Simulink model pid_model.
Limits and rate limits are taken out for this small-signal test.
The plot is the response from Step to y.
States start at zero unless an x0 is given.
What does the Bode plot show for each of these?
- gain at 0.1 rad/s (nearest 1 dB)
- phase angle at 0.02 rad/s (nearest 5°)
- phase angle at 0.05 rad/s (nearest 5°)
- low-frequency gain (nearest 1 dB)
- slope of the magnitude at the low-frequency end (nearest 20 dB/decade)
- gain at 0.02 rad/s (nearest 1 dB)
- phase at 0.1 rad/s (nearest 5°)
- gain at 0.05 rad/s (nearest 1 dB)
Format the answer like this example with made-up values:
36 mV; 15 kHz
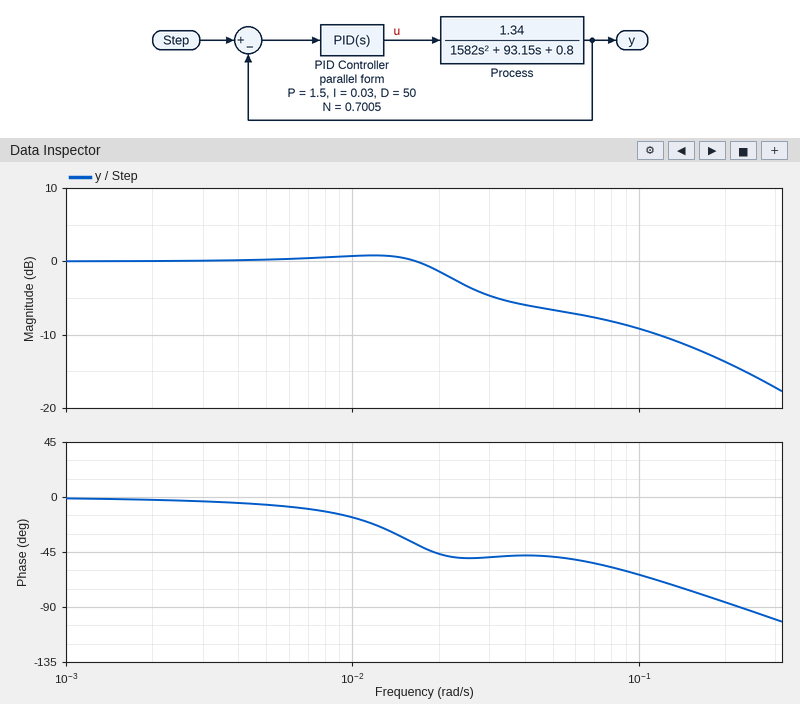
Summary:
-9 dB; -45°; -50°; 0 dB; 0 dB/decade; -1 dB; -65°; -7 dB
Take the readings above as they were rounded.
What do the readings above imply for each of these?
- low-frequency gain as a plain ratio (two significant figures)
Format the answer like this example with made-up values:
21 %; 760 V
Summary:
1.0
